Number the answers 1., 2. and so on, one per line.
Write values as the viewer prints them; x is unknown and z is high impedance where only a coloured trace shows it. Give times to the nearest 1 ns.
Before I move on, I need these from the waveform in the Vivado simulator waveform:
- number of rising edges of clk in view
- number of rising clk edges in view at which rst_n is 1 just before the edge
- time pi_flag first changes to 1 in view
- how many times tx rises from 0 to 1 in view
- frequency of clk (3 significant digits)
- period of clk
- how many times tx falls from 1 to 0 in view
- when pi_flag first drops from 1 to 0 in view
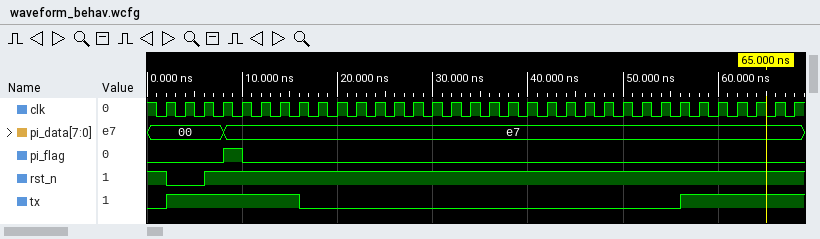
1. 34
2. 32
3. 8 ns
4. 2
5. 500 MHz
6. 2 ns
7. 1
8. 10 ns
